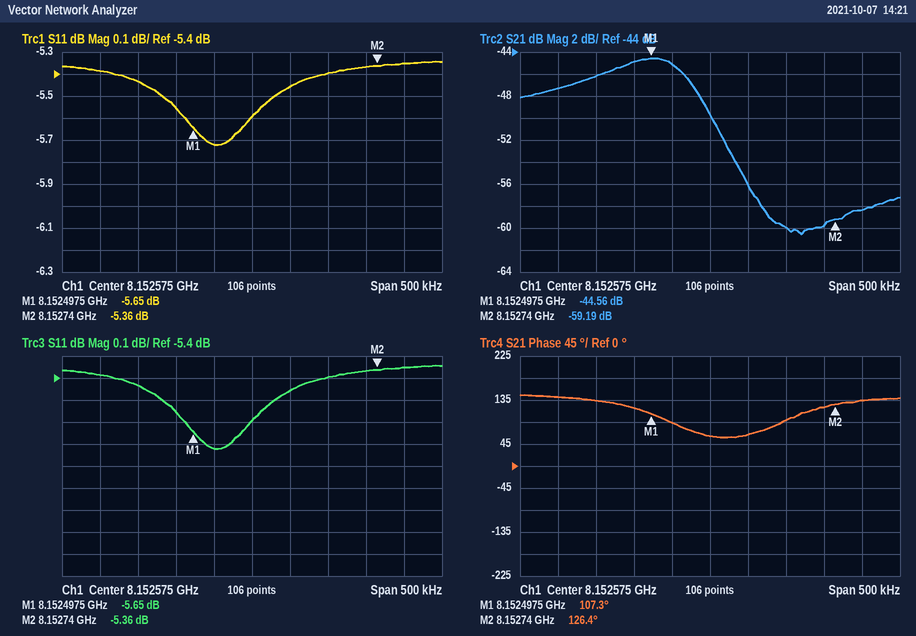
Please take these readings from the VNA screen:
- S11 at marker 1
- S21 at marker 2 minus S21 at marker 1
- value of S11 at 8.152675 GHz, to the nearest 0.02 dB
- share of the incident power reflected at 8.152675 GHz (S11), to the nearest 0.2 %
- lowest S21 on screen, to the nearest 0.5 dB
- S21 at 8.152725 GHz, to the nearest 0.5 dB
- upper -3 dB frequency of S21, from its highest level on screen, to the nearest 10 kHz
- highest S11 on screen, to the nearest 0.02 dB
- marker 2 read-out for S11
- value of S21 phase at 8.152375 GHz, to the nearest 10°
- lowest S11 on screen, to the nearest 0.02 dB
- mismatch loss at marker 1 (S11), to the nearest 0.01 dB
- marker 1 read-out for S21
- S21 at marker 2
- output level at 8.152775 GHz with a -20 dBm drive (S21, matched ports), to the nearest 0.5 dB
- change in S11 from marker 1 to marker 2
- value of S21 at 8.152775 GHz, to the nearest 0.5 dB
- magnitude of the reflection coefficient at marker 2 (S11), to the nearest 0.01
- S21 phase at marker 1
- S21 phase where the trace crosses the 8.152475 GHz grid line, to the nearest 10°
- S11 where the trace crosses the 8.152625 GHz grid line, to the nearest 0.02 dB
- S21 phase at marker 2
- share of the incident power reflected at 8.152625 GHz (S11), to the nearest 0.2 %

-5.65 dB
-14.63 dB
-5.40 dB
28.8 %
-60.5 dB
-60.0 dB
8.15256 GHz
-5.34 dB
-5.36 dB
140°
-5.72 dB
1.38 dB
-44.56 dB
-59.19 dB
-78.5 dBm
0.29 dB
-58.5 dB
0.54
107.3°
120°
-5.46 dB
126.4°
28.4 %
